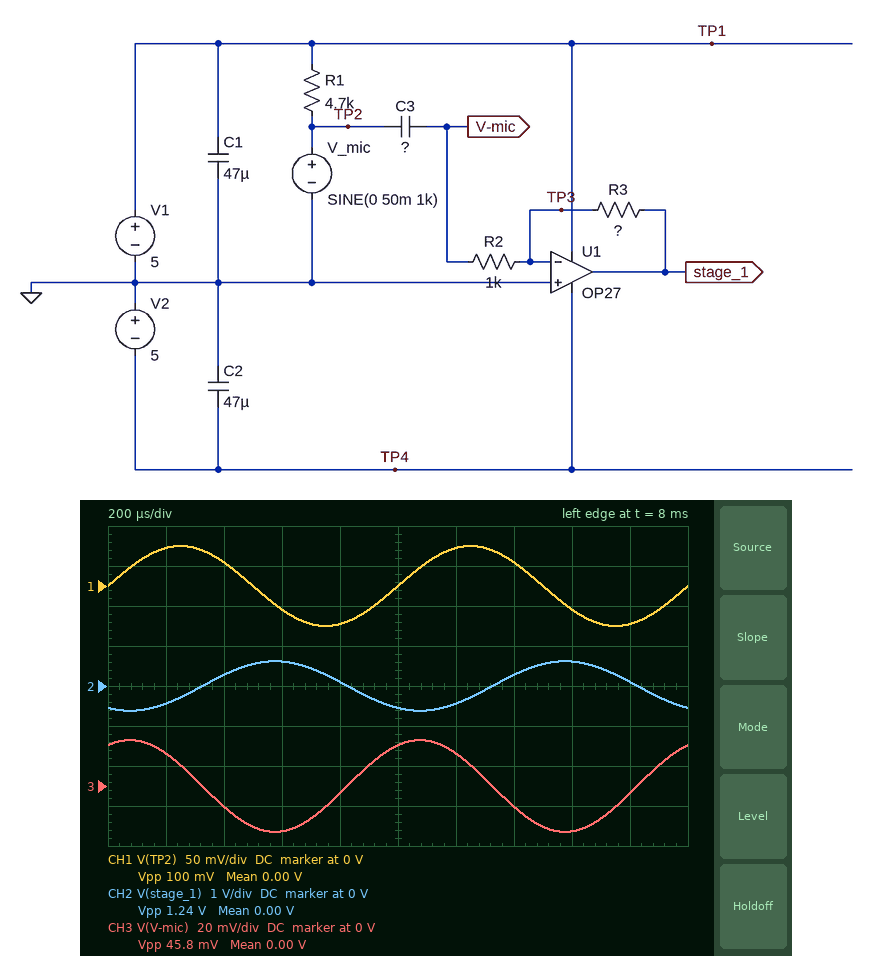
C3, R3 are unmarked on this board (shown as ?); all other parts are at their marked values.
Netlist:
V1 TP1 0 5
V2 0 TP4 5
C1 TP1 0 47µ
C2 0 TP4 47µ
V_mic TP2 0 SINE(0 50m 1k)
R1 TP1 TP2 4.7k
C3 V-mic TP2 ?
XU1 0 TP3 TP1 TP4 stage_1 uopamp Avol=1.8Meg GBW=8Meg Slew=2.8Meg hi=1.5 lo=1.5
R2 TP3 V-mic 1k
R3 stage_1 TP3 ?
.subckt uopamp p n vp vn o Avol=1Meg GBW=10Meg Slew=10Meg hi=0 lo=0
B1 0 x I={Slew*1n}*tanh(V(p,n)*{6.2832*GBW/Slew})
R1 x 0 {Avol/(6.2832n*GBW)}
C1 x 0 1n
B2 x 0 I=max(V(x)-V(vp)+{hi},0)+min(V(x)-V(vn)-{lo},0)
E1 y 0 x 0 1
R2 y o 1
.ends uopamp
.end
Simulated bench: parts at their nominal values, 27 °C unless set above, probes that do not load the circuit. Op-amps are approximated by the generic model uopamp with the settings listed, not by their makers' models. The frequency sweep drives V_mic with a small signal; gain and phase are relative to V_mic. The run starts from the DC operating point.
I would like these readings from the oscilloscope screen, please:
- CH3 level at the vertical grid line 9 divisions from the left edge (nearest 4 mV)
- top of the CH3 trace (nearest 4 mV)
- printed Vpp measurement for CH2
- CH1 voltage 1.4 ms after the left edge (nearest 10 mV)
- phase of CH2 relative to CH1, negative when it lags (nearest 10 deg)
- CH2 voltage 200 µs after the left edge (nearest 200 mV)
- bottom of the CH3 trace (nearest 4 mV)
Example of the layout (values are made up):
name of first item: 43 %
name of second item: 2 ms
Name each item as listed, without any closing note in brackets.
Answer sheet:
CH3 level at the vertical grid line 9 divisions from the left edge: -4 mV
top of the CH3 trace: 24 mV
printed Vpp measurement for CH2: 1.24 V
CH1 voltage 1.4 ms after the left edge: 30 mV
phase of CH2 relative to CH1, negative when it lags: -120 deg
CH2 voltage 200 µs after the left edge: -400 mV
bottom of the CH3 trace: -24 mV
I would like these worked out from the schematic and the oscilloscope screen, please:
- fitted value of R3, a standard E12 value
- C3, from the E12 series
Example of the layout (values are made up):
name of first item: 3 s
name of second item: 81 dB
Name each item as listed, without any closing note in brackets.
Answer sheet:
fitted value of R3, a standard E12 value: 27 kΩ
C3, from the E12 series: 82 nF
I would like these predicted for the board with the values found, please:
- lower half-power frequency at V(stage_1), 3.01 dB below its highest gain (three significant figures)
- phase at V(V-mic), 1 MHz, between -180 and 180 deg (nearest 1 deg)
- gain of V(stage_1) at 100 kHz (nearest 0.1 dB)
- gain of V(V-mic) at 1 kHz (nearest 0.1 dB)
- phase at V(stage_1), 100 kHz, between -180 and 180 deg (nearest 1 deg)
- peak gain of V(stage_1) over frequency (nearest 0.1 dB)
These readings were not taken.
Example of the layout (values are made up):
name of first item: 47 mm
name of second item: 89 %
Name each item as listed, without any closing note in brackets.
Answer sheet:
lower half-power frequency at V(stage_1), 3.01 dB below its highest gain: 1.93 kHz
phase at V(V-mic), 1 MHz, between -180 and 180 deg: 0 deg
gain of V(stage_1) at 100 kHz: 28.2 dB
gain of V(V-mic) at 1 kHz: -6.8 dB
phase at V(stage_1), 100 kHz, between -180 and 180 deg: 162 deg
peak gain of V(stage_1) over frequency: 28.6 dB
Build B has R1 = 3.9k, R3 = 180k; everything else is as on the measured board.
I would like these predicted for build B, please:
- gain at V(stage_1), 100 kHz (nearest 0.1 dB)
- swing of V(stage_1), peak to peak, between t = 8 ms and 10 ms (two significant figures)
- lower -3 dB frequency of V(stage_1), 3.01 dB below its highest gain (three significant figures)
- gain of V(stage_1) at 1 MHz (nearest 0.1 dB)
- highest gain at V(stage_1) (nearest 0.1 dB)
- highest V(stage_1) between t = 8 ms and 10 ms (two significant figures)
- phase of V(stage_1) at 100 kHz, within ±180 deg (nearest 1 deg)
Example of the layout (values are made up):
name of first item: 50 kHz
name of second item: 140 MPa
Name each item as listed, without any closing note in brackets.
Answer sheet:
gain at V(stage_1), 100 kHz: 37.3 dB
swing of V(stage_1), peak to peak, between t = 8 ms and 10 ms: 7.0 V
lower -3 dB frequency of V(stage_1), 3.01 dB below its highest gain: 1.86 kHz
gain of V(stage_1) at 1 MHz: 18.0 dB
highest gain at V(stage_1): 45.1 dB
highest V(stage_1) between t = 8 ms and 10 ms: 3.5 V
phase of V(stage_1) at 100 kHz, within ±180 deg: 114 deg
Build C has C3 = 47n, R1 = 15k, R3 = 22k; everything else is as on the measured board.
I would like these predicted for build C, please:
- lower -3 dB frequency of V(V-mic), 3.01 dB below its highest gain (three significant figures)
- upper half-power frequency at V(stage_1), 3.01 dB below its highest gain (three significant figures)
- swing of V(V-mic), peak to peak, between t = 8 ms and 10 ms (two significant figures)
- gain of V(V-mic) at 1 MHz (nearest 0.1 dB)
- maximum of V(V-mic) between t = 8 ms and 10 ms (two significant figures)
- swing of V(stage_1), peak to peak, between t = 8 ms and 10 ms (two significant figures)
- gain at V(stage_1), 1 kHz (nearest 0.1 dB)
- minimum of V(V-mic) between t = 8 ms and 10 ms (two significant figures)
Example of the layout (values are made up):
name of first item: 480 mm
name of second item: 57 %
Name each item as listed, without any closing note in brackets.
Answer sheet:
lower -3 dB frequency of V(V-mic), 3.01 dB below its highest gain: 3.41 kHz
upper half-power frequency at V(stage_1), 3.01 dB below its highest gain: 351 kHz
swing of V(V-mic), peak to peak, between t = 8 ms and 10 ms: 28 mV
gain of V(V-mic) at 1 MHz: 0 dB
maximum of V(V-mic) between t = 8 ms and 10 ms: 14 mV
swing of V(stage_1), peak to peak, between t = 8 ms and 10 ms: 620 mV
gain at V(stage_1), 1 kHz: 15.9 dB
minimum of V(V-mic) between t = 8 ms and 10 ms: -14 mV
